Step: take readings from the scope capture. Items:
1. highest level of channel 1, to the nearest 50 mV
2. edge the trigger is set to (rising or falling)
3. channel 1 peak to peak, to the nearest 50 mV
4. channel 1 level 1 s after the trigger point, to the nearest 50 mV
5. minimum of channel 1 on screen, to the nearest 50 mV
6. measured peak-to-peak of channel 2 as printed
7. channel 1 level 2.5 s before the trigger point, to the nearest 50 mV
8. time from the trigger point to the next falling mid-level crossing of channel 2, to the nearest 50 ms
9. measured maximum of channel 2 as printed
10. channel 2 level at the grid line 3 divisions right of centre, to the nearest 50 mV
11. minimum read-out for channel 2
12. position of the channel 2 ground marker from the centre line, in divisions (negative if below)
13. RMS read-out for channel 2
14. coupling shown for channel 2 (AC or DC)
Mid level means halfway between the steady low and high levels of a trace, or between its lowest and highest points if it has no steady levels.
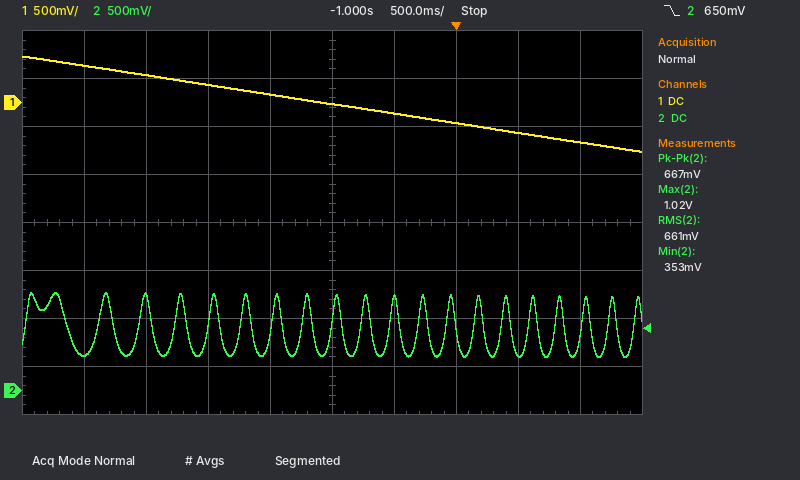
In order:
500 mV
falling
1.00 V
-400 mV
-500 mV
667 mV
300 mV
200 ms
1.02 V
400 mV
353 mV
-3.5 div
661 mV
DC
